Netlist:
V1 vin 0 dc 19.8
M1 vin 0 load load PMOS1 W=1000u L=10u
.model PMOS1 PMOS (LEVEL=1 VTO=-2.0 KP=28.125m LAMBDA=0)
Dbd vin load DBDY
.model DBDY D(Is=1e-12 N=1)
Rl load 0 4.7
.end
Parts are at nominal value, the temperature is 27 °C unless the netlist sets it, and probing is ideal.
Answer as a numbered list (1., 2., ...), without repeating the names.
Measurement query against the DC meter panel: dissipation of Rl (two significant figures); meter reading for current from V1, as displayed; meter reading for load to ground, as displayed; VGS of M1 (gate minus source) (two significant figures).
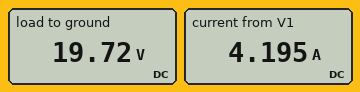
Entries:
1. 83 W
2. 4.195 A
3. 19.72 V
4. -20 V
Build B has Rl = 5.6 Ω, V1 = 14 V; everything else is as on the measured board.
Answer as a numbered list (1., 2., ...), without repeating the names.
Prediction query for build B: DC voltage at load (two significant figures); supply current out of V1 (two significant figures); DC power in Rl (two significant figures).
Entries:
1. 14 V
2. 2.5 A
3. 35 W
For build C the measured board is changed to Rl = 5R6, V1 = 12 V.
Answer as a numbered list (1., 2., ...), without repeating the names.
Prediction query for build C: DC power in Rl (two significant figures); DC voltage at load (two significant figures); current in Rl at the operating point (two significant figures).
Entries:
1. 25 W
2. 12 V
3. 2.1 A
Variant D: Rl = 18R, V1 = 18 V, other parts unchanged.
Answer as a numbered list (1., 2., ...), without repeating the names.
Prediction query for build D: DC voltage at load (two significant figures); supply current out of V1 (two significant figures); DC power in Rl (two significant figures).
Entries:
1. 18 V
2. 1.0 A
3. 18 W
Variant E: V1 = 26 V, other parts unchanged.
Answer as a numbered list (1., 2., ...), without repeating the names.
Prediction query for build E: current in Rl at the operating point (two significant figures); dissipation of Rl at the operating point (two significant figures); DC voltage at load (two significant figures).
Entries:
1. 5.5 A
2. 140 W
3. 26 V
